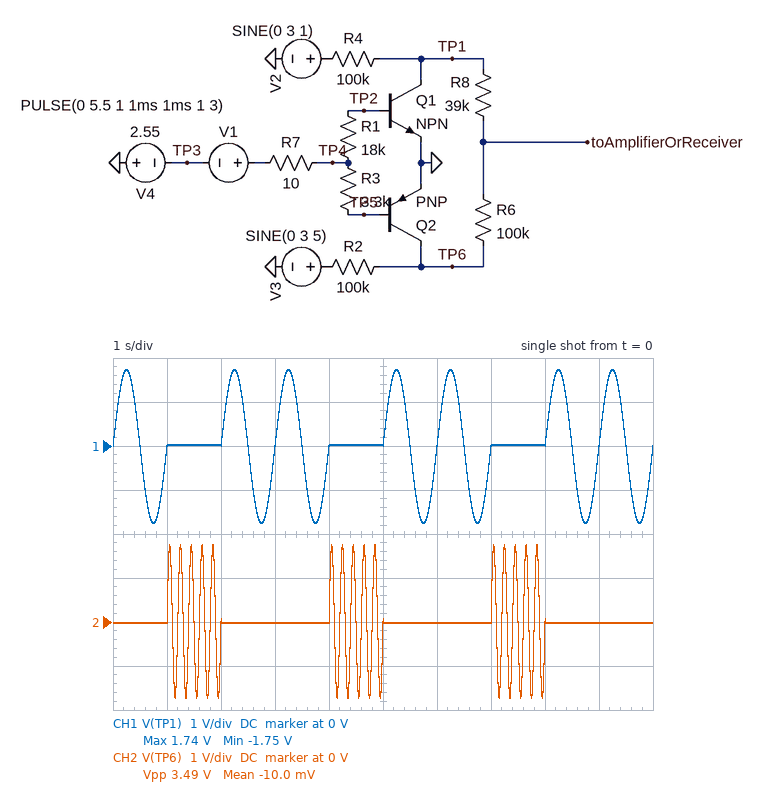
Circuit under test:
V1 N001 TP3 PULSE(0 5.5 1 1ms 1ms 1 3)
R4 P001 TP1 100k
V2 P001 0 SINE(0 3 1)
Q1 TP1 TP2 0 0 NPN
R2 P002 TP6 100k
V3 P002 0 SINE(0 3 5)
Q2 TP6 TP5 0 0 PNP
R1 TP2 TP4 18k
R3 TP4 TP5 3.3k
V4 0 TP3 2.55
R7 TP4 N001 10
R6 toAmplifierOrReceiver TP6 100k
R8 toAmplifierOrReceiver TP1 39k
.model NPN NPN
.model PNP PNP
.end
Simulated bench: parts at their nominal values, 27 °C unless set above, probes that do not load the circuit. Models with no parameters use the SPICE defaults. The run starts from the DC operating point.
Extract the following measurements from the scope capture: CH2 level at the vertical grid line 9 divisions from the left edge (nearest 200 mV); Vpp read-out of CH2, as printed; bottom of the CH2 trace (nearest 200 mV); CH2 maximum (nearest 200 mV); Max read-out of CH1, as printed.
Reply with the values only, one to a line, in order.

0 V
3.49 V
-1.8 V
1.8 V
1.74 V
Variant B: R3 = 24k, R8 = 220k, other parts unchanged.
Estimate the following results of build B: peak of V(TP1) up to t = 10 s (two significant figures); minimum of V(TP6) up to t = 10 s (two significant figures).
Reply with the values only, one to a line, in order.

2.3 V
-2.3 V
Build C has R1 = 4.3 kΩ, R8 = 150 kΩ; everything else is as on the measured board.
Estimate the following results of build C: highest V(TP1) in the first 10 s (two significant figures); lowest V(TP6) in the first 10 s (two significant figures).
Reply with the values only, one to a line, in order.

2.1 V
-2.1 V
